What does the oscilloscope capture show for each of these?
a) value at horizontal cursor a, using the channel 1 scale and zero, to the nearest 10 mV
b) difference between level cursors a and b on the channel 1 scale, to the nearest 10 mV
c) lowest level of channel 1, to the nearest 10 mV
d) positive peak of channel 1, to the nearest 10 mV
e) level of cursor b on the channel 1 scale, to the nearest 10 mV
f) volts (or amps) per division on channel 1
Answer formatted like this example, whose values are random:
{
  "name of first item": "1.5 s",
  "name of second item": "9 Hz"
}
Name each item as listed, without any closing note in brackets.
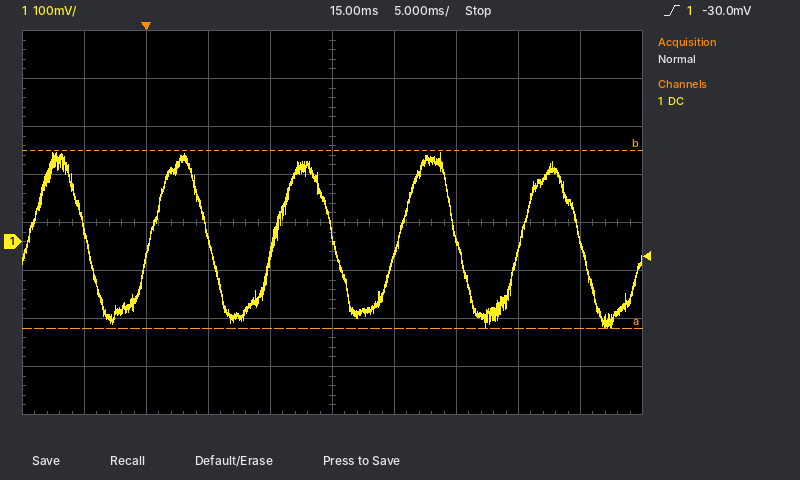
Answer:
{
  "value at horizontal cursor a, using the channel 1 scale and zero, to the nearest 10 mV": "-180 mV",
  "difference between level cursors a and b on the channel 1 scale, to the nearest 10 mV": "370 mV",
  "lowest level of channel 1, to the nearest 10 mV": "-180 mV",
  "positive peak of channel 1, to the nearest 10 mV": "190 mV",
  "level of cursor b on the channel 1 scale, to the nearest 10 mV": "190 mV",
  "volts (or amps) per division on channel 1": "100 mV"
}
